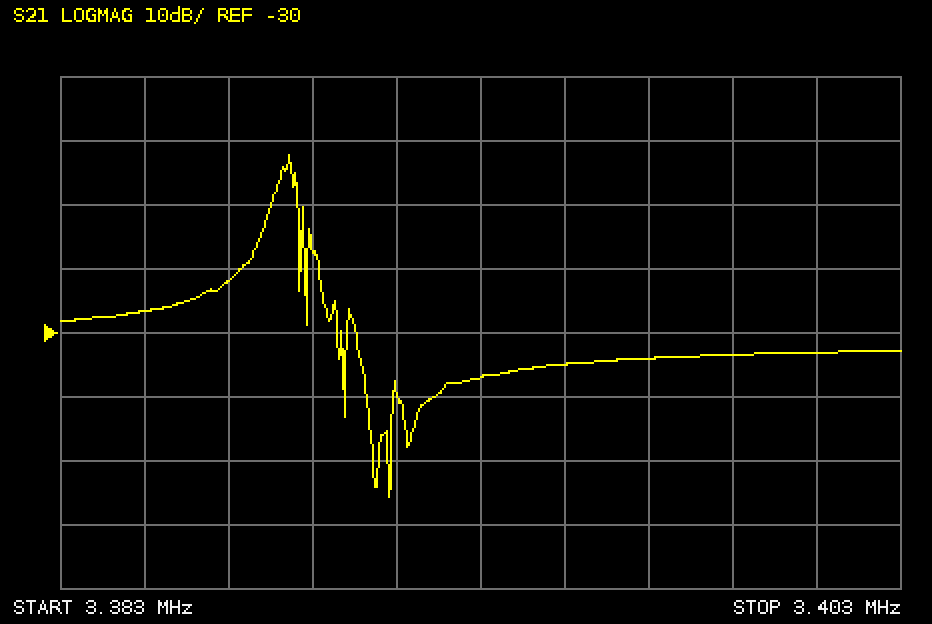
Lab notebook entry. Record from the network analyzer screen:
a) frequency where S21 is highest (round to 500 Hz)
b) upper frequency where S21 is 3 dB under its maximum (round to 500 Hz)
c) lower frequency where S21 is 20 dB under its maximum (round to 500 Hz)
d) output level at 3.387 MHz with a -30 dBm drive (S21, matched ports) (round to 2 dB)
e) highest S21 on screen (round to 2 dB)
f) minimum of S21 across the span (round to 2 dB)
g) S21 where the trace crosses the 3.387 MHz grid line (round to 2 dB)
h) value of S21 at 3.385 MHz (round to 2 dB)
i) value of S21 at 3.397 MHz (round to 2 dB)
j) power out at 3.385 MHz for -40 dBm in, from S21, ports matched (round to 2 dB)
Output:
3.3885 MHz
3.3885 MHz
3.3870 MHz
-52 dBm
-2 dB
-56 dB
-22 dB
-26 dB
-34 dB
-66 dBm
